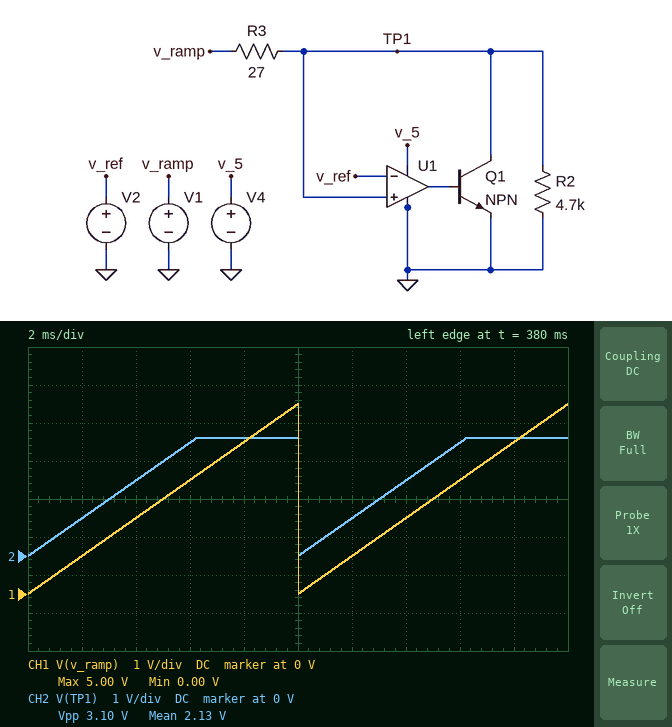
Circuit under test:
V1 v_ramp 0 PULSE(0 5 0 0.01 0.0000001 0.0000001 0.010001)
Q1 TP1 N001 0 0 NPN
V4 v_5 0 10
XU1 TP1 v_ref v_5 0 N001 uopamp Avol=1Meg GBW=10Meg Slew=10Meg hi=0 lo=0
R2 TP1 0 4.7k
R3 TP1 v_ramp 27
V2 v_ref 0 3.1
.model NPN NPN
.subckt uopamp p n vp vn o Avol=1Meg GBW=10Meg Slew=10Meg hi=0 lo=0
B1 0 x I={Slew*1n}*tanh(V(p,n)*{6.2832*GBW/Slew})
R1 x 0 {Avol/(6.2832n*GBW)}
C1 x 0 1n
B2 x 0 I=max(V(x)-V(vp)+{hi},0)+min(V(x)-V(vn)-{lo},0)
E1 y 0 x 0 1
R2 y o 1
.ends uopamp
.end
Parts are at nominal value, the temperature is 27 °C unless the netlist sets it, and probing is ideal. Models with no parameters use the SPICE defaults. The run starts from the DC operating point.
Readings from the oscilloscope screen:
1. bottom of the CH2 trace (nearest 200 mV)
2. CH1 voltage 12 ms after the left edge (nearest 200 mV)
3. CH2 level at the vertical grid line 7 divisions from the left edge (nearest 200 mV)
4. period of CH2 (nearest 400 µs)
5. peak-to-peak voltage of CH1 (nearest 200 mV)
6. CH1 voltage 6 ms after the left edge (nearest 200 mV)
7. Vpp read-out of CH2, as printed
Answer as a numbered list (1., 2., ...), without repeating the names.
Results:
1. 0 V
2. 1.0 V
3. 2.0 V
4. 10.0 ms
5. 5.0 V
6. 3.0 V
7. 3.10 V
